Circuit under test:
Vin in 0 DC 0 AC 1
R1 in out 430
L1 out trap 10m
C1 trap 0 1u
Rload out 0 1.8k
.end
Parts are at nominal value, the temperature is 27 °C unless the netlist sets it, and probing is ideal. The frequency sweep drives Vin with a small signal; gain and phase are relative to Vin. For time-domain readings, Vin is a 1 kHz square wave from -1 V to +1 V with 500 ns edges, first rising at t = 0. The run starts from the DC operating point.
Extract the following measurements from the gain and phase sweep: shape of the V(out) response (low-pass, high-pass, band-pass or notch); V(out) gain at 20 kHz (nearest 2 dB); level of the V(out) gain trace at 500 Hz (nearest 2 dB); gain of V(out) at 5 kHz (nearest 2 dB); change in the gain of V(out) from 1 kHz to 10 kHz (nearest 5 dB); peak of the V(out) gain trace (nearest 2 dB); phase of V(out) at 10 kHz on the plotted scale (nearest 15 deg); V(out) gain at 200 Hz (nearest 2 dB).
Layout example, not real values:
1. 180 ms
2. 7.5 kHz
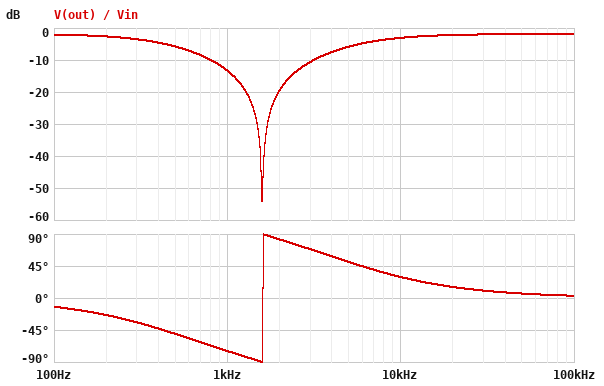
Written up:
1. notch
2. -2 dB
3. -6 dB
4. -6 dB
5. 10 dB
6. -2 dB
7. 30 deg
8. -2 dB
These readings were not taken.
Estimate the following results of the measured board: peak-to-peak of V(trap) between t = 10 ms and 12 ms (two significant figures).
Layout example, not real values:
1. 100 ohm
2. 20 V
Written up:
1. 1.0 V
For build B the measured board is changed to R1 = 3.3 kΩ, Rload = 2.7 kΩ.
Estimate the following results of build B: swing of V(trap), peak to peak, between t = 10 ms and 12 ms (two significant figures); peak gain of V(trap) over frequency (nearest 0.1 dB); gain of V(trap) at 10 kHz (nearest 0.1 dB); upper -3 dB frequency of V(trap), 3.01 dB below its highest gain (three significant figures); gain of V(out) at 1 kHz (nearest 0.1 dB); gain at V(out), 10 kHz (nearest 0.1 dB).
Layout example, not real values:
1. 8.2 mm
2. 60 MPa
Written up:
1. 150 mV
2. -6.9 dB
3. -47.0 dB
4. 108 Hz
5. -30.7 dB
6. -15.3 dB
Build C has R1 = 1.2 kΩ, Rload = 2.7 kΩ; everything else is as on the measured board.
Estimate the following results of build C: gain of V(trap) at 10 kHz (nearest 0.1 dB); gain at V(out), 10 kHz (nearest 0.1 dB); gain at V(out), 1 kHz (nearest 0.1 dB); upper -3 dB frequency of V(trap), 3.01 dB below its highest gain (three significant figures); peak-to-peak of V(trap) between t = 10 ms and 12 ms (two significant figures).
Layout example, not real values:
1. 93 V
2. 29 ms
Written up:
1. -39.4 dB
2. -7.7 dB
3. -22.0 dB
4. 194 Hz
5. 400 mV
